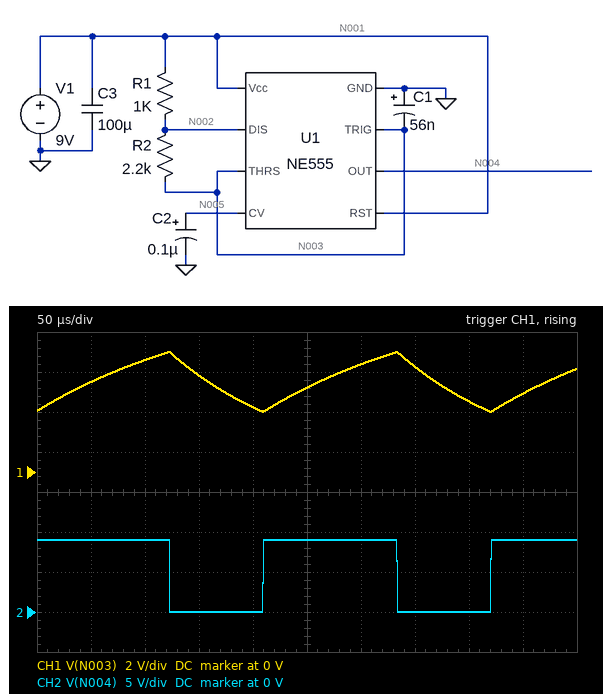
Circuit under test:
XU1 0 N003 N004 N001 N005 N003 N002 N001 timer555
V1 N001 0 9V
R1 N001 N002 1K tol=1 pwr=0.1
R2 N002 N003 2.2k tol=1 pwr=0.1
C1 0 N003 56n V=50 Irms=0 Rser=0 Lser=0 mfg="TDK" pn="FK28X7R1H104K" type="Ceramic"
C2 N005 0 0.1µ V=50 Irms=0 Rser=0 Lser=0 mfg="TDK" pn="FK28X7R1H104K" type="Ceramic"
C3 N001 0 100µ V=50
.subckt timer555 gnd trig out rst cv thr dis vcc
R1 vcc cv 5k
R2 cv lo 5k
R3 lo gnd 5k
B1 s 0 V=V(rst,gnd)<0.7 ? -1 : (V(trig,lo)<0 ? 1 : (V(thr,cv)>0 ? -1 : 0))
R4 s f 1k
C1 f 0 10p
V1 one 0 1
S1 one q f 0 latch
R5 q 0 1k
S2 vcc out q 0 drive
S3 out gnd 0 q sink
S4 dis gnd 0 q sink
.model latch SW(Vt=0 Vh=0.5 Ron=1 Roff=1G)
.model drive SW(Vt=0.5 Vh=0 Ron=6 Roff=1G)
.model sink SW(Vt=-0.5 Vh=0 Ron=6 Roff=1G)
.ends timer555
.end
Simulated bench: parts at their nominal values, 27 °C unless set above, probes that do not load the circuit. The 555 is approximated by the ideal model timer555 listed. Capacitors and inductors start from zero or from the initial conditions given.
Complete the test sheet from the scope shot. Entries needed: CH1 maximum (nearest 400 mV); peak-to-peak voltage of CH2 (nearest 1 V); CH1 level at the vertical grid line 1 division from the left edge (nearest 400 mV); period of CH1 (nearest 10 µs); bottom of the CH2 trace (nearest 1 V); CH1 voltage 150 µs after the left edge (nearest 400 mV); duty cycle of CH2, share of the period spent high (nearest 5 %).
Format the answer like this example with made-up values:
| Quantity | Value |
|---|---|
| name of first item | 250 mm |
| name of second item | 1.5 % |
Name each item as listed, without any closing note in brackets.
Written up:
| Quantity | Value |
|---|---|
| CH1 maximum | 6.0 V |
| peak-to-peak voltage of CH2 | 9 V |
| CH1 level at the vertical grid line 1 division from the left edge | 4.4 V |
| period of CH1 | 210 µs |
| bottom of the CH2 trace | 0 V |
| CH1 voltage 150 µs after the left edge | 4.8 V |
| duty cycle of CH2, share of the period spent high | 60 % |
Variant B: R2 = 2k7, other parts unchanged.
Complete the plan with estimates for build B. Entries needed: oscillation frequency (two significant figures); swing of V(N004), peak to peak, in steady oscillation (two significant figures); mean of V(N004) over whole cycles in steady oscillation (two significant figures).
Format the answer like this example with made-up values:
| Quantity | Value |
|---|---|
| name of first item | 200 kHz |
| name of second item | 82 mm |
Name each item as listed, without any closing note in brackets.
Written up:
| Quantity | Value |
|---|---|
| oscillation frequency | 4.0 kHz |
| swing of V(N004), peak to peak, in steady oscillation | 9.0 V |
| mean of V(N004) over whole cycles in steady oscillation | 5.2 V |
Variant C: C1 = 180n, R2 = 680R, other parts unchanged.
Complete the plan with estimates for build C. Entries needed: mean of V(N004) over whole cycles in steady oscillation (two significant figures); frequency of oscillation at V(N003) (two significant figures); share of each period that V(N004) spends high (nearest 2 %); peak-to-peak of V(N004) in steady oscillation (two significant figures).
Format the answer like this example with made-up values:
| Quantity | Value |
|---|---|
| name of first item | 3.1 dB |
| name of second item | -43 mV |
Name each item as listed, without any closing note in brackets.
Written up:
| Quantity | Value |
|---|---|
| mean of V(N004) over whole cycles in steady oscillation | 6.4 V |
| frequency of oscillation at V(N003) | 3.4 kHz |
| share of each period that V(N004) spends high | 70 % |
| peak-to-peak of V(N004) in steady oscillation | 9.0 V |
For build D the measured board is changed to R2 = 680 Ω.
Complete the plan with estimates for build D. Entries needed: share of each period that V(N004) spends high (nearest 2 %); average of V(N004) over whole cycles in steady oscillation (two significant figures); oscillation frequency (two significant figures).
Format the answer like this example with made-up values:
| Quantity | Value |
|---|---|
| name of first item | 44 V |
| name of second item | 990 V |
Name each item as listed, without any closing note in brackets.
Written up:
| Quantity | Value |
|---|---|
| share of each period that V(N004) spends high | 70 % |
| average of V(N004) over whole cycles in steady oscillation | 6.4 V |
| oscillation frequency | 11 kHz |
